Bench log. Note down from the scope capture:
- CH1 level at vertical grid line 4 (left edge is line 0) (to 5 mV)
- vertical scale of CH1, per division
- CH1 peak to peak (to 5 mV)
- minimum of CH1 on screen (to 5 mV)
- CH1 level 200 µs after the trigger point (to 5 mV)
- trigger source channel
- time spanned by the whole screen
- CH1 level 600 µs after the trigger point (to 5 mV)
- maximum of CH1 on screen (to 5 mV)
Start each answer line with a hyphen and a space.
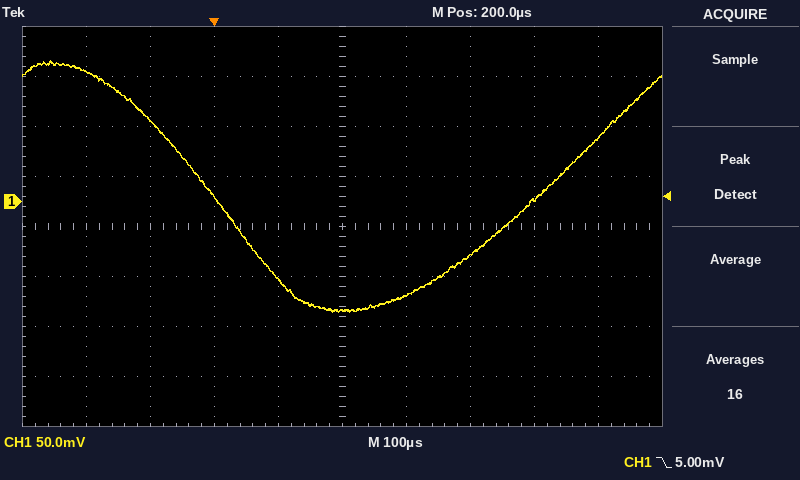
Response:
- -80 mV
- 50 mV
- 250 mV
- -110 mV
- -110 mV
- CH1
- 1 ms
- 65 mV
- 140 mV
